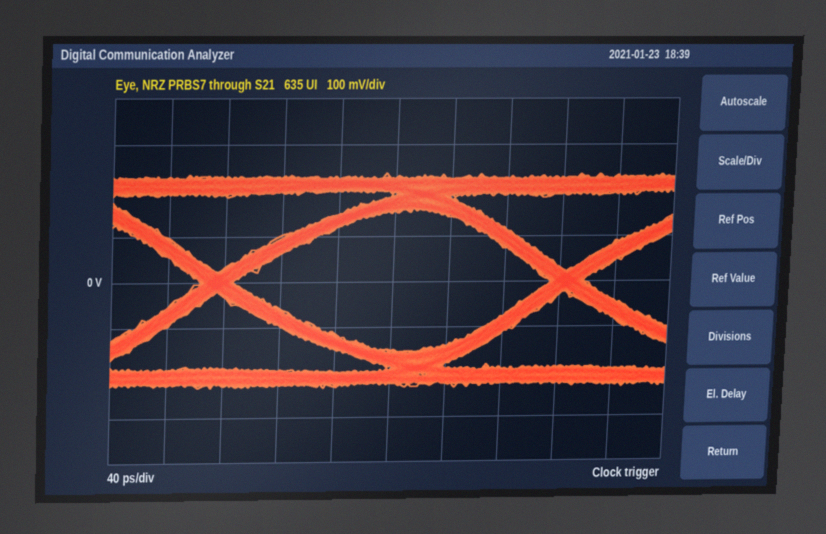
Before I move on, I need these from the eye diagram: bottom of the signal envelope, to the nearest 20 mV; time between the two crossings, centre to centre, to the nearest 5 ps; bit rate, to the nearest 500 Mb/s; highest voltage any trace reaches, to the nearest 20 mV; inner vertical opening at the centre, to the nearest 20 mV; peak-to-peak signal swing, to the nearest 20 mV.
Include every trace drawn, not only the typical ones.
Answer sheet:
-240 mV
250 ps
4.0 Gb/s
240 mV
300 mV
480 mV
